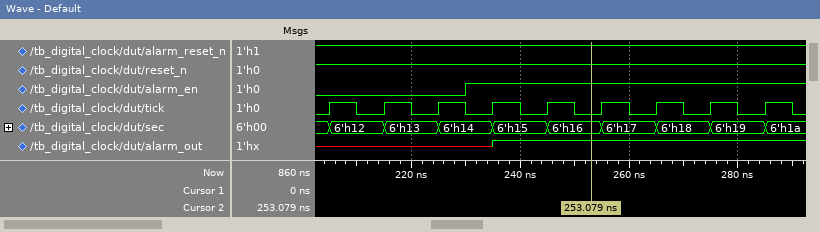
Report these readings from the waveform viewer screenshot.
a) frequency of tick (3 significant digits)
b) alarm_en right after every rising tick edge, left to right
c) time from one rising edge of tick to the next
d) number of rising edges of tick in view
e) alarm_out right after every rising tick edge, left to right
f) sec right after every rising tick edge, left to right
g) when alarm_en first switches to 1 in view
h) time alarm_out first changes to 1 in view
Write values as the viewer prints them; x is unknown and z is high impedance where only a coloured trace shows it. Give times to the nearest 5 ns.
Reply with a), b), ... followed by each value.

a) 100 MHz
b) 0 0 0 1 1 1 1 1 1
c) 10 ns
d) 9
e) x x x 1 1 1 1 1 1
f) 6'h12, 6'h13, 6'h14, 6'h15, 6'h16, 6'h17, 6'h18, 6'h19, 6'h1a
g) 230 ns
h) 235 ns
